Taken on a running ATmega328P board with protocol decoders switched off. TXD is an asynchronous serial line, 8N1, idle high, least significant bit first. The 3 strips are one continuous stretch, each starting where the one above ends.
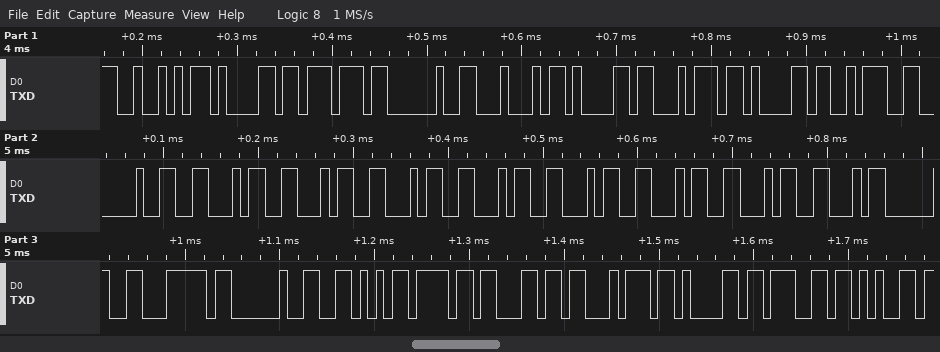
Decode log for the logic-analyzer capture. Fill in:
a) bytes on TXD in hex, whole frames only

0x52 0x61 0x77 0x20 0x44 0x61 0x74 0x61 0x3A 0x20 0x46 0x46 0x46 0x46 0x46 0x46 0x46 0x46 0x20 0x7C 0x20 0x56 0x6F 0x6C 0x74 0x61 0x67 0x65
